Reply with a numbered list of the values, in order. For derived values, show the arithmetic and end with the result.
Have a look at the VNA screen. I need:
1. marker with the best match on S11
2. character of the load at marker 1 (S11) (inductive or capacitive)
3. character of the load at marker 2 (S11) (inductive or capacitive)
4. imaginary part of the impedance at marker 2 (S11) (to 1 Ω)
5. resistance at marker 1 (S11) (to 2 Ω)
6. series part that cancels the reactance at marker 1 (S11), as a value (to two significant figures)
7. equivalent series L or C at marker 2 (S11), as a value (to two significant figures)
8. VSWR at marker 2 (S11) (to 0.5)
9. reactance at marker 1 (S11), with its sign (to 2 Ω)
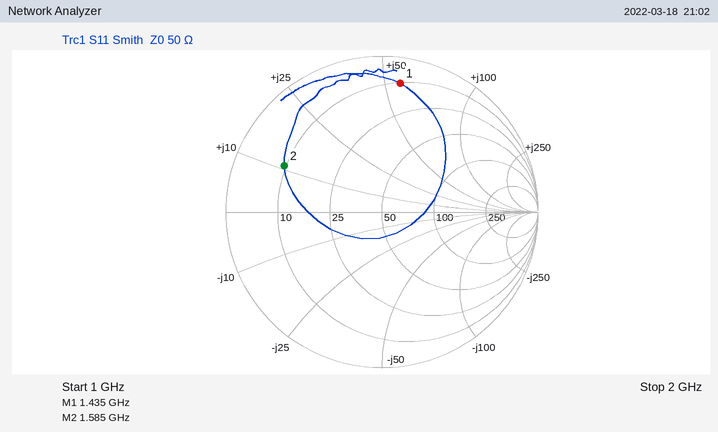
1. marker 2
2. inductive
3. inductive
4. +11 Ω
5. 10 Ω
6. C = 1/(2π × 1.435 GHz × 56 Ω) ≈ 2.0 pF
7. L = 11 Ω/(2π × 1.585 GHz) ≈ 1.1 nH
8. 5.5
9. +56 Ω
